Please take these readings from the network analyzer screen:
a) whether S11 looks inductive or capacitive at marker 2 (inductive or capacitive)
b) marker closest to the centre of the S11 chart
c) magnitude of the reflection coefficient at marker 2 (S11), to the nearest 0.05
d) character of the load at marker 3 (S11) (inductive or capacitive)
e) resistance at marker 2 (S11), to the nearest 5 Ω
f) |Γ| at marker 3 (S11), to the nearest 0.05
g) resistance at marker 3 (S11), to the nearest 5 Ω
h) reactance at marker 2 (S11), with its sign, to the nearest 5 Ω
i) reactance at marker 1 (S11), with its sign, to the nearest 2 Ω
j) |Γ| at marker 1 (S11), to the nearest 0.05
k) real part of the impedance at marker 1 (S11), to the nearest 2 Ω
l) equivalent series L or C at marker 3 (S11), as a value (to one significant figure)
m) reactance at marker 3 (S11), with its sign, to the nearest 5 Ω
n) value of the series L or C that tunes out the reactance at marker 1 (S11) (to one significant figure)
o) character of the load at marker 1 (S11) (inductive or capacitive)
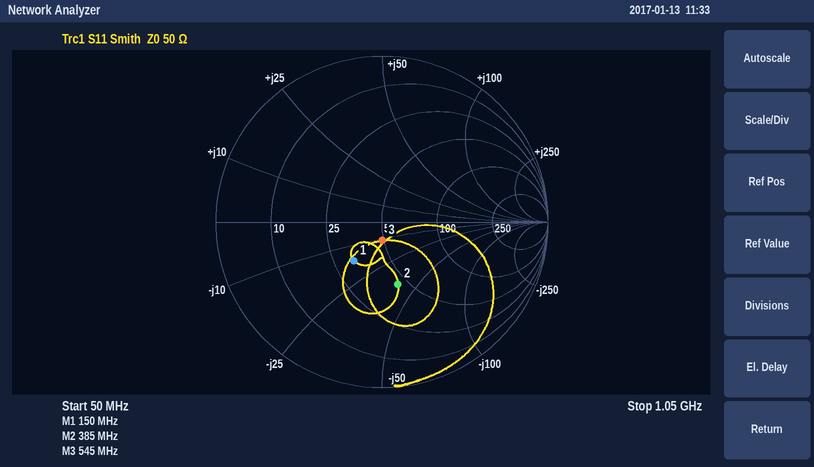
capacitive
marker 3
0.40
capacitive
45 Ω
0.10
50 Ω
-40 Ω
-16 Ω
0.30
32 Ω
30 pF
-10 Ω
20 nH
capacitive
